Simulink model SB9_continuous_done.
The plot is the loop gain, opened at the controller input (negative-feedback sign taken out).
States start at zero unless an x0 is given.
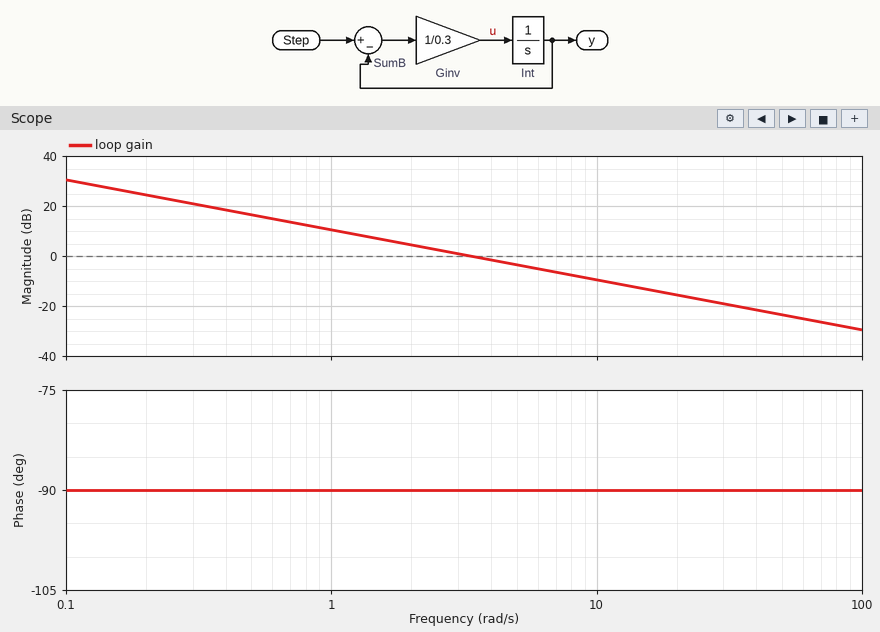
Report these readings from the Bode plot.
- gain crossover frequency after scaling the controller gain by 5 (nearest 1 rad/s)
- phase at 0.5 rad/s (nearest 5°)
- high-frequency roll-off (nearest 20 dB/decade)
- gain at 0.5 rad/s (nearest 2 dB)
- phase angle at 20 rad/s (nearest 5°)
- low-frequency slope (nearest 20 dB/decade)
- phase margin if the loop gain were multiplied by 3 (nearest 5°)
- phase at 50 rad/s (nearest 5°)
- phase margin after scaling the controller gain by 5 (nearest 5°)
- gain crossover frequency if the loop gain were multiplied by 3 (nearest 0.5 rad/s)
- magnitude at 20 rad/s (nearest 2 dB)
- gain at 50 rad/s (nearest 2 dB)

17 rad/s
-90°
-20 dB/decade
16 dB
-90°
-20 dB/decade
90°
-90°
90°
10.0 rad/s
-16 dB
-24 dB
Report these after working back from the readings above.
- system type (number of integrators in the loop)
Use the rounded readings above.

1
